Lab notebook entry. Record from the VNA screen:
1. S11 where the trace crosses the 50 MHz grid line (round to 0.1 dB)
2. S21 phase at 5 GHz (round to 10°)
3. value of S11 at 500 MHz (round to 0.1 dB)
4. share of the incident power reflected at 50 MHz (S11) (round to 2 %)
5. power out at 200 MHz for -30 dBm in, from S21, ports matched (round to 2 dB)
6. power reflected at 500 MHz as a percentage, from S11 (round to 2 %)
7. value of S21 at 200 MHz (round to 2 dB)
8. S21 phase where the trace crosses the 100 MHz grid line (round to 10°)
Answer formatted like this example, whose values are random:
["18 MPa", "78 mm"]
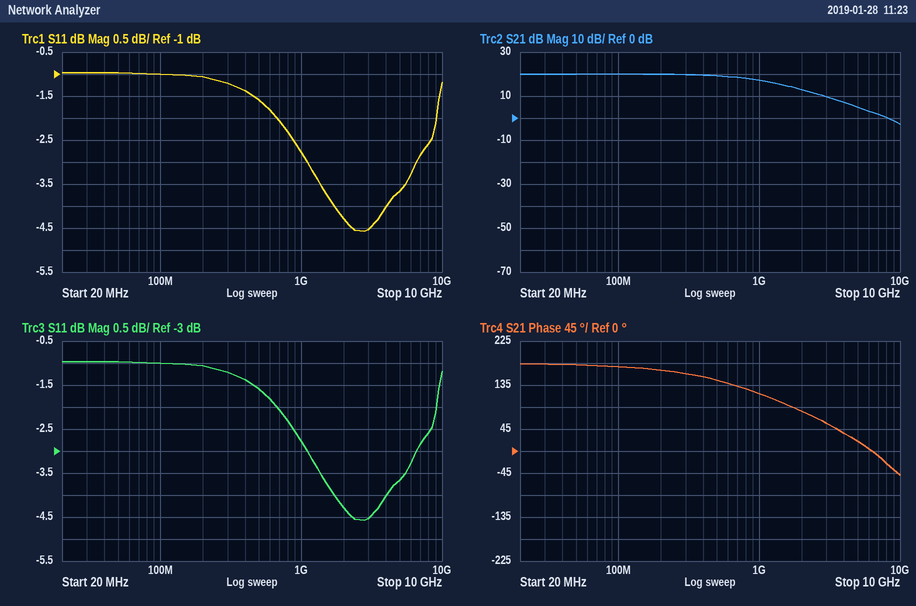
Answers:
["-1.0 dB", "20°", "-1.6 dB", "80 %", "-10 dBm", "70 %", "20 dB", "170°"]
